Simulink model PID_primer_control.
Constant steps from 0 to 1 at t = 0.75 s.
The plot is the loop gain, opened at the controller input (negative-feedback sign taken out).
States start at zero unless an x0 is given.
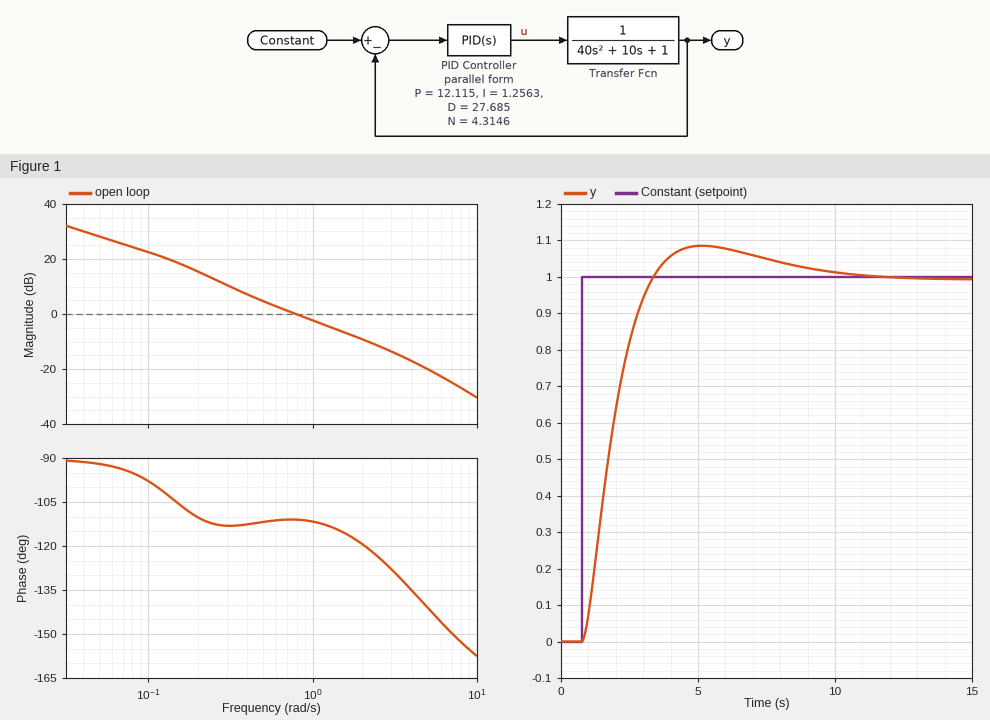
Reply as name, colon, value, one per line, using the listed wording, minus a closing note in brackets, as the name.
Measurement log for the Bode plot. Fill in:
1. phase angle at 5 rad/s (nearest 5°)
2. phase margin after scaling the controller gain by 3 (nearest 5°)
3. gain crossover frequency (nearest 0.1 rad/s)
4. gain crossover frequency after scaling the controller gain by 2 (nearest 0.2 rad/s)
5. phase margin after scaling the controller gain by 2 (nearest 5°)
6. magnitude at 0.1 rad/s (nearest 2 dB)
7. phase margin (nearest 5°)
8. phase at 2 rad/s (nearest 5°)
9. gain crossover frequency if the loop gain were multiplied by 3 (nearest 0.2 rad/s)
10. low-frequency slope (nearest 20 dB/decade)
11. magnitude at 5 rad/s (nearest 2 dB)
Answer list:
phase angle at 5 rad/s: -140°
phase margin after scaling the controller gain by 3: 60°
gain crossover frequency: 0.8 rad/s
gain crossover frequency after scaling the controller gain by 2: 1.4 rad/s
phase margin after scaling the controller gain by 2: 65°
magnitude at 0.1 rad/s: 22 dB
phase margin: 70°
phase at 2 rad/s: -120°
gain crossover frequency if the loop gain were multiplied by 3: 2.0 rad/s
low-frequency slope: -20 dB/decade
magnitude at 5 rad/s: -20 dB
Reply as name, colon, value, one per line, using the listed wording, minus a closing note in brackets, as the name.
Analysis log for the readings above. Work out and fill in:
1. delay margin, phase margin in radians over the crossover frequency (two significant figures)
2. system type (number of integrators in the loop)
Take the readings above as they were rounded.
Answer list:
delay margin, phase margin in radians over the crossover frequency: 1.5 s
system type: 1
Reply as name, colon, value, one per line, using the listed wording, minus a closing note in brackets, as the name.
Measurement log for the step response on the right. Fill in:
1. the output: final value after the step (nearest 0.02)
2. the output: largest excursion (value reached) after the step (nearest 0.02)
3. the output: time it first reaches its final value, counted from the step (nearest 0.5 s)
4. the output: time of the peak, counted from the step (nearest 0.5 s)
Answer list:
the output: final value after the step: 1.00
the output: largest excursion (value reached) after the step: 1.08
the output: time it first reaches its final value, counted from the step: 2.5 s
the output: time of the peak, counted from the step: 4.5 s
